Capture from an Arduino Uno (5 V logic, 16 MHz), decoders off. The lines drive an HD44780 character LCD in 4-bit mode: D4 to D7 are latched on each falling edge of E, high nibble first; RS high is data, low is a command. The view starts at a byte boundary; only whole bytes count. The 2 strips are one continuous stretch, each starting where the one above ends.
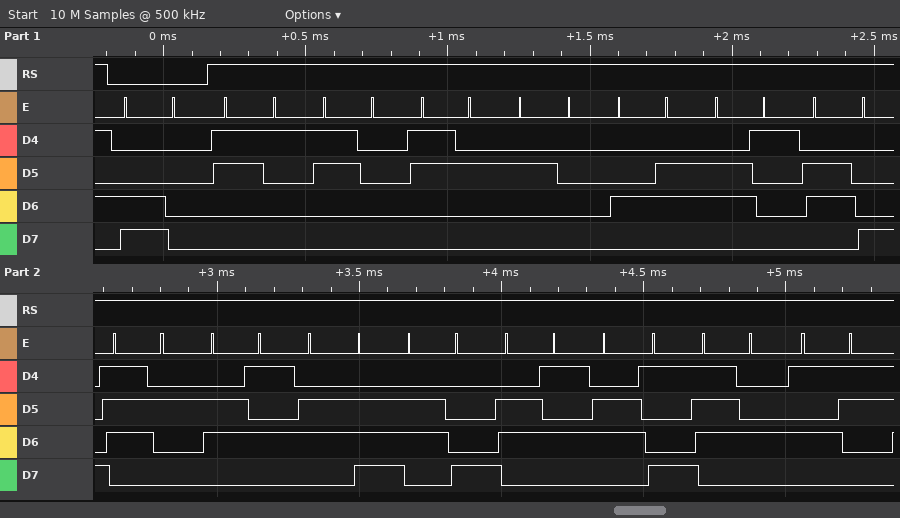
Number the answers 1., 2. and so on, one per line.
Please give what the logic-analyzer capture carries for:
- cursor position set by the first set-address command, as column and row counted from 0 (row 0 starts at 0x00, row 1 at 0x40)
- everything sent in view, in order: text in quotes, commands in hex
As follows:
1. column 0, row 1
2. 0xC0 "102 FahrenheitS"
